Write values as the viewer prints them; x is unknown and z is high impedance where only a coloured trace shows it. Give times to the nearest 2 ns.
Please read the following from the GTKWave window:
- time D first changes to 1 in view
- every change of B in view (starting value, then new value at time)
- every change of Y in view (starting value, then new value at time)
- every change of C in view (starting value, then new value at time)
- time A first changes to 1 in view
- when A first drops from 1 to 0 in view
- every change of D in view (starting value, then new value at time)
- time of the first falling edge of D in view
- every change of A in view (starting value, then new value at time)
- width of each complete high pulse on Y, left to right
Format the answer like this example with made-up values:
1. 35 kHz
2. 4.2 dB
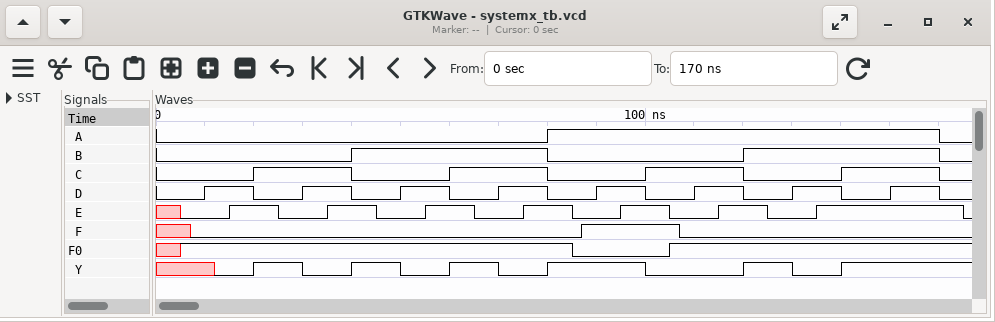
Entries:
1. 10 ns
2. 0, 1 at 40 ns, 0 at 80 ns, 1 at 120 ns, 0 at 160 ns
3. x, 0 at 12 ns, 1 at 20 ns, 0 at 30 ns, 1 at 40 ns, 0 at 50 ns, 1 at 60 ns, 0 at 70 ns, 1 at 80 ns, 0 at 100 ns, 1 at 120 ns, 0 at 130 ns, 1 at 140 ns
4. 0, 1 at 20 ns, 0 at 40 ns, 1 at 60 ns, 0 at 80 ns, 1 at 100 ns, 0 at 120 ns, 1 at 140 ns, 0 at 160 ns
5. 80 ns
6. 160 ns
7. 0, 1 at 10 ns, 0 at 20 ns, 1 at 30 ns, 0 at 40 ns, 1 at 50 ns, 0 at 60 ns, 1 at 70 ns, 0 at 80 ns, 1 at 90 ns, 0 at 100 ns, 1 at 110 ns, 0 at 120 ns, 1 at 130 ns, 0 at 140 ns, 1 at 150 ns, 0 at 160 ns
8. 20 ns
9. 0, 1 at 80 ns, 0 at 160 ns
10. 10 ns, 10 ns, 10 ns, 20 ns, 10 ns
